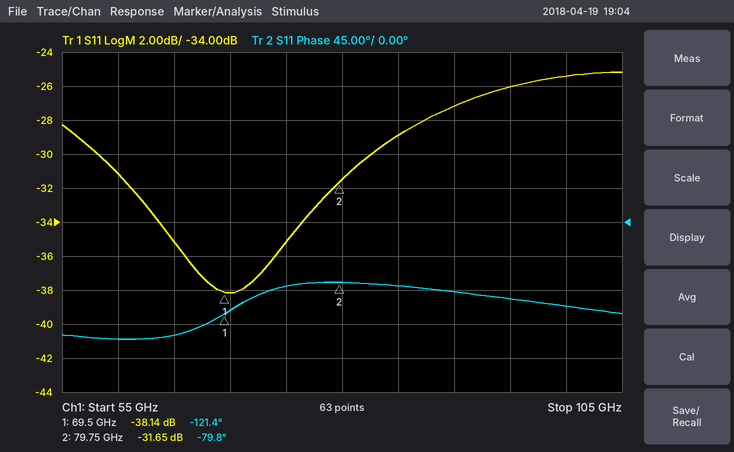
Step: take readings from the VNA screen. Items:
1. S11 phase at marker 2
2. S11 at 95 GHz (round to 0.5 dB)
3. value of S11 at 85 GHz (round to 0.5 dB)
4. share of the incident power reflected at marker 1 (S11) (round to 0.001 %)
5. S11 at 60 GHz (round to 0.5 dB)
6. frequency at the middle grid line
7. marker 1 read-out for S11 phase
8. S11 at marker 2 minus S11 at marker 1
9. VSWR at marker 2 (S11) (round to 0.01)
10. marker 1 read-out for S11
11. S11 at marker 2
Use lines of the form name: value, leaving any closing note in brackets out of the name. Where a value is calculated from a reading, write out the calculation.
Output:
S11 phase at marker 2: -79.8°
S11 at 95 GHz: -26.0 dB
value of S11 at 85 GHz: -29.0 dB
share of the incident power reflected at marker 1 (S11): 10^(-38.14/10) ≈ 0.015 %
S11 at 60 GHz: -31.0 dB
frequency at the middle grid line: 80 GHz
marker 1 read-out for S11 phase: -121.4°
S11 at marker 2 minus S11 at marker 1: -31.65 − (-38.14) = 6.49 dB
VSWR at marker 2 (S11): (1 + 0.0262)/(1 − 0.0262) ≈ 1.05
marker 1 read-out for S11: -38.14 dB
S11 at marker 2: -31.65 dB
